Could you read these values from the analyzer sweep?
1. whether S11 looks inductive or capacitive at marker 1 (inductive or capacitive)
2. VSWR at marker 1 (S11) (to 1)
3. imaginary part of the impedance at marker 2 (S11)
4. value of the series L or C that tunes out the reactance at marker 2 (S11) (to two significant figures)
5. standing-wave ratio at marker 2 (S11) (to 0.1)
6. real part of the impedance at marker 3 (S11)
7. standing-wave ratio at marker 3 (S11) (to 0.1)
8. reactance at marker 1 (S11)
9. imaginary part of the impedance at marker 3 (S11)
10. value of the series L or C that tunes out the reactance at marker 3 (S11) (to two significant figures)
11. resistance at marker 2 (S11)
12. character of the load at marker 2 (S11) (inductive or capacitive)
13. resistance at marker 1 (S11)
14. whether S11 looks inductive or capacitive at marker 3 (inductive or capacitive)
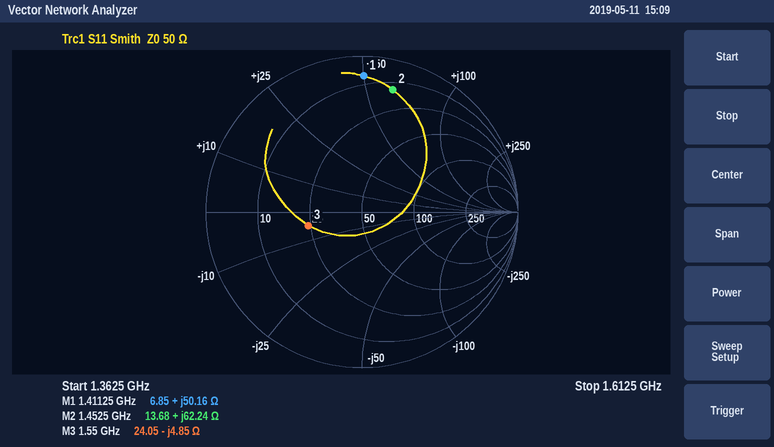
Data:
inductive
15
+62.24 Ω
1.8 pF
9.5
24.05 Ω
2.1
+50.16 Ω
-4.85 Ω
500 pH
13.68 Ω
inductive
6.85 Ω
capacitive
